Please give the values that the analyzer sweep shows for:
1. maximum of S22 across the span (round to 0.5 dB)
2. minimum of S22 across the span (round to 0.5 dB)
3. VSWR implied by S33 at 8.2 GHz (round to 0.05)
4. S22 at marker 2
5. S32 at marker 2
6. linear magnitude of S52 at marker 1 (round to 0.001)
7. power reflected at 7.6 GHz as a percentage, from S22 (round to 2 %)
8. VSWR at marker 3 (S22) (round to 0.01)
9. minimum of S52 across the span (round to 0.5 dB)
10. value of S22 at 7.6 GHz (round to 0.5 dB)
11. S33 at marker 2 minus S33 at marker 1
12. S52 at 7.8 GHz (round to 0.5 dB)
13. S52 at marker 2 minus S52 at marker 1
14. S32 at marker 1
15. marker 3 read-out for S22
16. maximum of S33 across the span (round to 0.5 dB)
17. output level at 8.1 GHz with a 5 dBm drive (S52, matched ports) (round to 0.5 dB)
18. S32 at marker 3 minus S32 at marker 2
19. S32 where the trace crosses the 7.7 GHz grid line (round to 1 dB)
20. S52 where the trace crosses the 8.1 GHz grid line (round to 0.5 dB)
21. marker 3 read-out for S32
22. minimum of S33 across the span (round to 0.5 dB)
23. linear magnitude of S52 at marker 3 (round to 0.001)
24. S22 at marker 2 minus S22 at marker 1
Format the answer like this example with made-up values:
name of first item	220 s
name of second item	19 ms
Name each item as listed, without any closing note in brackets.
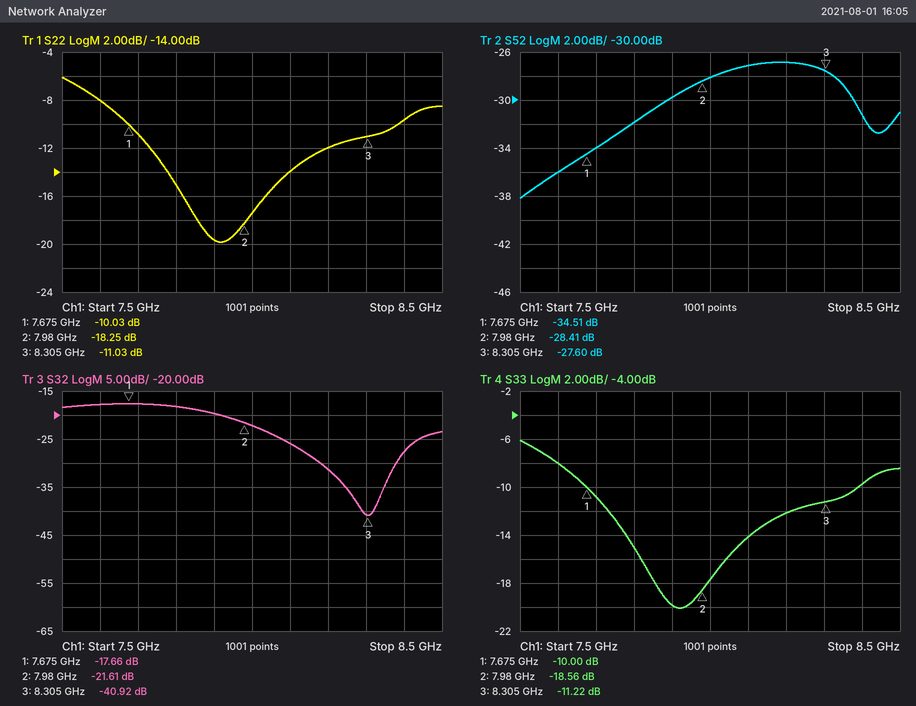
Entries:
maximum of S22 across the span	-6.0 dB
minimum of S22 across the span	-20.0 dB
VSWR implied by S33 at 8.2 GHz	1.65
S22 at marker 2	-18.25 dB
S32 at marker 2	-21.61 dB
linear magnitude of S52 at marker 1	0.019
power reflected at 7.6 GHz as a percentage, from S22	16 %
VSWR at marker 3 (S22)	1.78
minimum of S52 across the span	-38.0 dB
value of S22 at 7.6 GHz	-8.0 dB
S33 at marker 2 minus S33 at marker 1	-8.56 dB
S52 at 7.8 GHz	-32.0 dB
S52 at marker 2 minus S52 at marker 1	6.10 dB
S32 at marker 1	-17.66 dB
marker 3 read-out for S22	-11.03 dB
maximum of S33 across the span	-6.0 dB
output level at 8.1 GHz with a 5 dBm drive (S52, matched ports)	-22.0 dBm
S32 at marker 3 minus S32 at marker 2	-19.31 dB
S32 where the trace crosses the 7.7 GHz grid line	-18 dB
S52 where the trace crosses the 8.1 GHz grid line	-27.0 dB
marker 3 read-out for S32	-40.92 dB
minimum of S33 across the span	-20.0 dB
linear magnitude of S52 at marker 3	0.042
S22 at marker 2 minus S22 at marker 1	-8.22 dB
